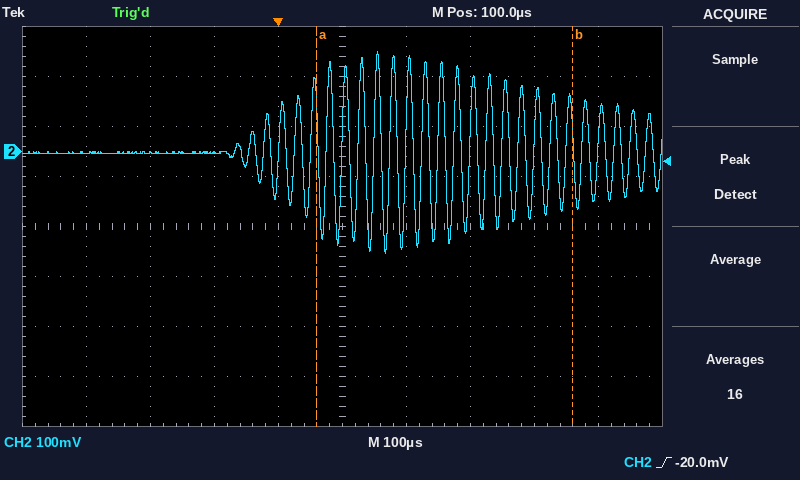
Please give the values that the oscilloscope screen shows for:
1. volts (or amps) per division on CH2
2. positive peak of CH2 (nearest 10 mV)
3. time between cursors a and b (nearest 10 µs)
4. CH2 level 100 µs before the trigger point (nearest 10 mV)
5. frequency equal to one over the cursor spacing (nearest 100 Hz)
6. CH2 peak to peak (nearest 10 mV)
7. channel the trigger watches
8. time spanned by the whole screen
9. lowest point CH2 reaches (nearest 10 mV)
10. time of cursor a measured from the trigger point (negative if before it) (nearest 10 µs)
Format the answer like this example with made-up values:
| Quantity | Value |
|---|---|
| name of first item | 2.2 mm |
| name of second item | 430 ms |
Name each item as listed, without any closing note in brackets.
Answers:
| Quantity | Value |
|---|---|
| volts (or amps) per division on CH2 | 100 mV |
| positive peak of CH2 | 200 mV |
| time between cursors a and b | 400 µs |
| CH2 level 100 µs before the trigger point | 0 mV |
| frequency equal to one over the cursor spacing | 2.5 kHz |
| CH2 peak to peak | 400 mV |
| channel the trigger watches | CH2 |
| time spanned by the whole screen | 1 ms |
| lowest point CH2 reaches | -200 mV |
| time of cursor a measured from the trigger point (negative if before it) | +60 µs |
